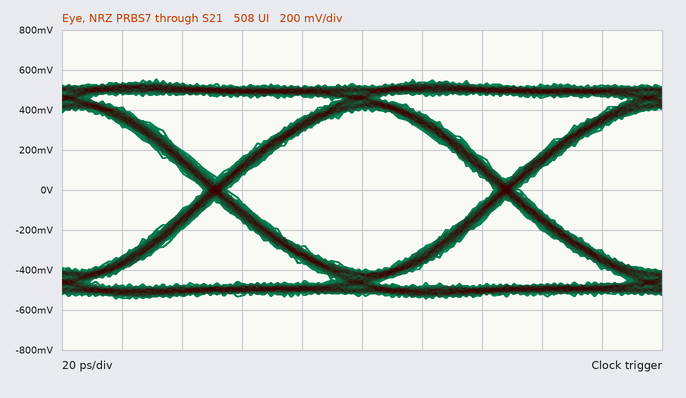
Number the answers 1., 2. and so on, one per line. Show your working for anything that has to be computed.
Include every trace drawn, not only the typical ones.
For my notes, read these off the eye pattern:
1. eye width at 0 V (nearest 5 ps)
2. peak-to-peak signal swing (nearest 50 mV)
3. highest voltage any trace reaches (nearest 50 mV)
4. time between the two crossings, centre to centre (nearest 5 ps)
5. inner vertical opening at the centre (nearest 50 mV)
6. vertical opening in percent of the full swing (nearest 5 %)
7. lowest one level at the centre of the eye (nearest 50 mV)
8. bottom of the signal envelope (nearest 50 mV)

1. 90 ps
2. 1.10 V
3. 550 mV
4. 95 ps
5. 800 mV
6. 800 mV / 1.10 V ≈ 72.7 %, so 75 % to the nearest 5 %
7. 400 mV
8. -550 mV
